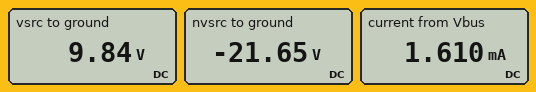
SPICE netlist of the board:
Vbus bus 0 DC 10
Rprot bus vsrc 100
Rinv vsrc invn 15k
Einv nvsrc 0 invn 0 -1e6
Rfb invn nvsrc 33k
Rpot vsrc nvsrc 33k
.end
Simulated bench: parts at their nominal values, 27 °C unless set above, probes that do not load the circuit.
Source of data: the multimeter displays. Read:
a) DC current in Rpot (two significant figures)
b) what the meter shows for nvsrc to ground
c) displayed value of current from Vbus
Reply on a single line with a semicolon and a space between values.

950 µA; -21.65 V; 1.610 mA
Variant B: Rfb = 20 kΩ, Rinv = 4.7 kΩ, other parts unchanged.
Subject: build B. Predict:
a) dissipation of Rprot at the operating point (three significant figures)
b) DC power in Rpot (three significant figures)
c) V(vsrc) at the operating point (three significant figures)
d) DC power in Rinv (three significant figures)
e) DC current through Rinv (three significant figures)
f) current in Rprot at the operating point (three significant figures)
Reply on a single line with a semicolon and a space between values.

1.29 mW; 77.8 mW; 9.64 V; 19.8 mW; 2.05 mA; 3.59 mA
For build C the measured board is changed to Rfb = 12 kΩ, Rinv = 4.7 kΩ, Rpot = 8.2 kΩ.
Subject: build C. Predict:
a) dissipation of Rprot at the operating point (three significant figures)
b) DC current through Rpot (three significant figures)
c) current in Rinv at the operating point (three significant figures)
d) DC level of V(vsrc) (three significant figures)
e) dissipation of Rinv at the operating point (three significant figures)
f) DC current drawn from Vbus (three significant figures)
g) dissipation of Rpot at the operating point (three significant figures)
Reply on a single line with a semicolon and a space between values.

3.68 mW; 4.07 mA; 2.00 mA; 9.39 V; 18.8 mW; 6.07 mA; 136 mW
